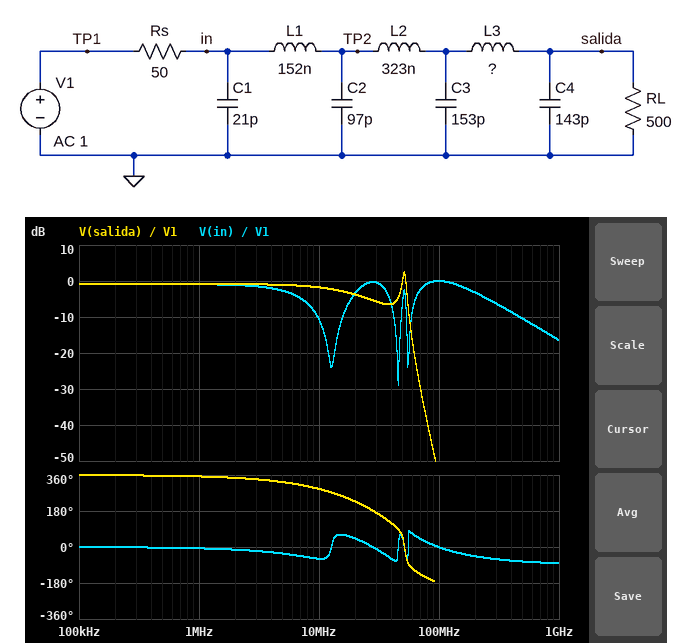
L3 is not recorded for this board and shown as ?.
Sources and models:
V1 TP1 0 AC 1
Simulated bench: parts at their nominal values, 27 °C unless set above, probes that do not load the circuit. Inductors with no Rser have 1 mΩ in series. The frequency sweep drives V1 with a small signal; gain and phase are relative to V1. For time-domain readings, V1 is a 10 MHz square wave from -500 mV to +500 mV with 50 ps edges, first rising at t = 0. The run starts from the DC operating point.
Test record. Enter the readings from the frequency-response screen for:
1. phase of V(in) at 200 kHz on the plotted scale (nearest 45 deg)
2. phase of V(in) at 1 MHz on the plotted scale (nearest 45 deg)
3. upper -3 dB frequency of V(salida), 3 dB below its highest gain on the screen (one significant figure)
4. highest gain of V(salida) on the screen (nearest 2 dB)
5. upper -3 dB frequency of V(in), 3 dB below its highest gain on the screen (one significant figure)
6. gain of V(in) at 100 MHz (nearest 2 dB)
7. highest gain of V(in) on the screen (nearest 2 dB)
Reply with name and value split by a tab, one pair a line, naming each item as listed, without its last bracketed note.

phase of V(in) at 200 kHz on the plotted scale	0 deg
phase of V(in) at 1 MHz on the plotted scale	0 deg
upper -3 dB frequency of V(salida), 3 dB below its highest gain on the screen	50 MHz
highest gain of V(salida) on the screen	2 dB
upper -3 dB frequency of V(in), 3 dB below its highest gain on the screen	200 MHz
gain of V(in) at 100 MHz	0 dB
highest gain of V(in) on the screen	0 dB
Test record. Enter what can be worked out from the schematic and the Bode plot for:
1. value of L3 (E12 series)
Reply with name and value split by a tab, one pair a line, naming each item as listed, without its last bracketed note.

value of L3	150 nH
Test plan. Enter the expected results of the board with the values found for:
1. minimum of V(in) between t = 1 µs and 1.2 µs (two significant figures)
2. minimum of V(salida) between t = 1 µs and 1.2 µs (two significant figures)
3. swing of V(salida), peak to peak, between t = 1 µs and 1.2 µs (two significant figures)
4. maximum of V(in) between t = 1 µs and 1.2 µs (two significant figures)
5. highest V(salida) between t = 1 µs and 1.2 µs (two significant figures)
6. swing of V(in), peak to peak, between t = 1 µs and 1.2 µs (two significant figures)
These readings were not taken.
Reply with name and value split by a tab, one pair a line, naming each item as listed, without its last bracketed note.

minimum of V(in) between t = 1 µs and 1.2 µs	-450 mV
minimum of V(salida) between t = 1 µs and 1.2 µs	-540 mV
swing of V(salida), peak to peak, between t = 1 µs and 1.2 µs	1.1 V
maximum of V(in) between t = 1 µs and 1.2 µs	450 mV
highest V(salida) between t = 1 µs and 1.2 µs	540 mV
swing of V(in), peak to peak, between t = 1 µs and 1.2 µs	900 mV
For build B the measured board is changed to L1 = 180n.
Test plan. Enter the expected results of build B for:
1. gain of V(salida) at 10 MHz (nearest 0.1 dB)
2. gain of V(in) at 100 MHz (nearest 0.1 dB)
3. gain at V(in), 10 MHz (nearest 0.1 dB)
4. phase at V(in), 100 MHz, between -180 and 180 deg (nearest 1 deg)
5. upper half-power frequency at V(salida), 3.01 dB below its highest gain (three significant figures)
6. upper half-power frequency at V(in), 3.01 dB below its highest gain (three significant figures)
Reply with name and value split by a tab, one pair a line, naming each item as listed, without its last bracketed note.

gain of V(salida) at 10 MHz	-1.7 dB
gain of V(in) at 100 MHz	-0.1 dB
gain at V(in), 10 MHz	-11.5 dB
phase at V(in), 100 MHz, between -180 and 180 deg	-8 deg
upper half-power frequency at V(salida), 3.01 dB below its highest gain	53.4 MHz
upper half-power frequency at V(in), 3.01 dB below its highest gain	189 MHz
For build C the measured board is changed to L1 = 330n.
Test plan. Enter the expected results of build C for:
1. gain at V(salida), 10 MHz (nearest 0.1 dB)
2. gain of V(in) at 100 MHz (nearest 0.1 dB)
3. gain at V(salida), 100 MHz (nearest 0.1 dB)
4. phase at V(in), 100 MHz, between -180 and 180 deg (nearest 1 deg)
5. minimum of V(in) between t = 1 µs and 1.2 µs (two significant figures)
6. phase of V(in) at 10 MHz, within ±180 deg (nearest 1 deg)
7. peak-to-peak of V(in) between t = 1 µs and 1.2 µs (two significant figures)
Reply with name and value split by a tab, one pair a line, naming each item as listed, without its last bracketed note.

gain at V(salida), 10 MHz	-1.3 dB
gain of V(in) at 100 MHz	-0.6 dB
gain at V(salida), 100 MHz	-62.7 dB
phase at V(in), 100 MHz, between -180 and 180 deg	-22 deg
minimum of V(in) between t = 1 µs and 1.2 µs	-410 mV
phase of V(in) at 10 MHz, within ±180 deg	-44 deg
peak-to-peak of V(in) between t = 1 µs and 1.2 µs	820 mV
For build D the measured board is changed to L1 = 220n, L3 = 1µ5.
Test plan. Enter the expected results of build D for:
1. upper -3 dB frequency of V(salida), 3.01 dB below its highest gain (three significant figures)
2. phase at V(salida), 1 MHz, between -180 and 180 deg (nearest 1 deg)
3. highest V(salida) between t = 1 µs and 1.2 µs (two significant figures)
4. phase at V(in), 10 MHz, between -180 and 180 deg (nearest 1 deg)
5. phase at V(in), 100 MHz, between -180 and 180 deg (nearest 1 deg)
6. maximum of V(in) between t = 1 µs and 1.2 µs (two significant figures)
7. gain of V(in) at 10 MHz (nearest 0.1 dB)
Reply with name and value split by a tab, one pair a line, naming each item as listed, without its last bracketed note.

upper -3 dB frequency of V(salida), 3.01 dB below its highest gain	14.9 MHz
phase at V(salida), 1 MHz, between -180 and 180 deg	-8 deg
highest V(salida) between t = 1 µs and 1.2 µs	860 mV
phase at V(in), 10 MHz, between -180 and 180 deg	27 deg
phase at V(in), 100 MHz, between -180 and 180 deg	-14 deg
maximum of V(in) between t = 1 µs and 1.2 µs	650 mV
gain of V(in) at 10 MHz	-8.6 dB
